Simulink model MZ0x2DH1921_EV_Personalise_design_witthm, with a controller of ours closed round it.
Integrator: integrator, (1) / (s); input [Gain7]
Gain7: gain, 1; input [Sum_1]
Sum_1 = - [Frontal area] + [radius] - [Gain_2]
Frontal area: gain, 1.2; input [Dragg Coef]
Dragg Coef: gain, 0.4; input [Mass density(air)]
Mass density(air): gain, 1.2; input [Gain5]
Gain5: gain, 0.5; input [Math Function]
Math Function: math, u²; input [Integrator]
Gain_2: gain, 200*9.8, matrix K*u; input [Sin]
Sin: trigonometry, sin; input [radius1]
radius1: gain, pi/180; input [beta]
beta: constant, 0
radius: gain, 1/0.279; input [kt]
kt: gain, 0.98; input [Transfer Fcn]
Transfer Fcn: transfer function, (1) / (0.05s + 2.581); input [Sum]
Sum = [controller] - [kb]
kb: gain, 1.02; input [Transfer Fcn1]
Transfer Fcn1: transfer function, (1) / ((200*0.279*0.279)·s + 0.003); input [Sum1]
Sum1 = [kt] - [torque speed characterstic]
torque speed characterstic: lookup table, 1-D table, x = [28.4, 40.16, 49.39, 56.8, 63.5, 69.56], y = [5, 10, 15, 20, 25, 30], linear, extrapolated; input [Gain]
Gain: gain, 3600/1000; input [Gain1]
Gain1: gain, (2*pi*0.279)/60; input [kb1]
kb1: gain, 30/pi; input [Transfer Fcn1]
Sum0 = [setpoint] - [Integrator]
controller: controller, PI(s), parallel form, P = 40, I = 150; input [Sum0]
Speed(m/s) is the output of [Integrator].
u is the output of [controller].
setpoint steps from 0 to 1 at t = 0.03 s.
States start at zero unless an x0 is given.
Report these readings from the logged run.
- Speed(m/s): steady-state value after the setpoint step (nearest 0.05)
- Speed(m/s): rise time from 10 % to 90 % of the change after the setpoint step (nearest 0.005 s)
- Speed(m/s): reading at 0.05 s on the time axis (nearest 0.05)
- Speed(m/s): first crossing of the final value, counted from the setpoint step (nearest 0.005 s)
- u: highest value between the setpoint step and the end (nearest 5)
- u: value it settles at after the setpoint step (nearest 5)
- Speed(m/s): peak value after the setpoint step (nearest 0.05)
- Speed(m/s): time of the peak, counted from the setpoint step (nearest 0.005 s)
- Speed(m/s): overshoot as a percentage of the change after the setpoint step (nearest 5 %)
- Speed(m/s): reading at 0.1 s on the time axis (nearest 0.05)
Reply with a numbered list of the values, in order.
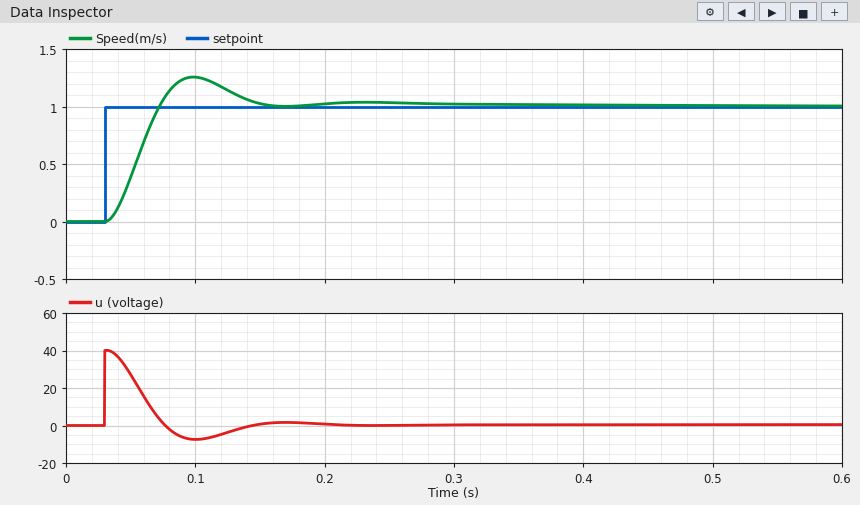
1. 1.00
2. 0.030 s
3. 0.40
4. 0.040 s
5. 40
6. 0
7. 1.25
8. 0.070 s
9. 25 %
10. 1.25
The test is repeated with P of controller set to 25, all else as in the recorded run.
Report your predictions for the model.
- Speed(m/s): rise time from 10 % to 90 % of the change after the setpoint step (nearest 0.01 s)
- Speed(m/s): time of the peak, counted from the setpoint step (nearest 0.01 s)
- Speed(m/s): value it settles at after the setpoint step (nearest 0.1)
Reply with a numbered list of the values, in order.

1. 0.04 s
2. 0.10 s
3. 1.0
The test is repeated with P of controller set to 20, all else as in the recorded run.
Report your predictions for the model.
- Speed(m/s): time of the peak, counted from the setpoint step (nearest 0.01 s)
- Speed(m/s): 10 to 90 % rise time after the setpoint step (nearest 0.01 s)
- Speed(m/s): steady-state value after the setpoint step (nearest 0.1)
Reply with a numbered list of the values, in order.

1. 0.11 s
2. 0.04 s
3. 1.0
